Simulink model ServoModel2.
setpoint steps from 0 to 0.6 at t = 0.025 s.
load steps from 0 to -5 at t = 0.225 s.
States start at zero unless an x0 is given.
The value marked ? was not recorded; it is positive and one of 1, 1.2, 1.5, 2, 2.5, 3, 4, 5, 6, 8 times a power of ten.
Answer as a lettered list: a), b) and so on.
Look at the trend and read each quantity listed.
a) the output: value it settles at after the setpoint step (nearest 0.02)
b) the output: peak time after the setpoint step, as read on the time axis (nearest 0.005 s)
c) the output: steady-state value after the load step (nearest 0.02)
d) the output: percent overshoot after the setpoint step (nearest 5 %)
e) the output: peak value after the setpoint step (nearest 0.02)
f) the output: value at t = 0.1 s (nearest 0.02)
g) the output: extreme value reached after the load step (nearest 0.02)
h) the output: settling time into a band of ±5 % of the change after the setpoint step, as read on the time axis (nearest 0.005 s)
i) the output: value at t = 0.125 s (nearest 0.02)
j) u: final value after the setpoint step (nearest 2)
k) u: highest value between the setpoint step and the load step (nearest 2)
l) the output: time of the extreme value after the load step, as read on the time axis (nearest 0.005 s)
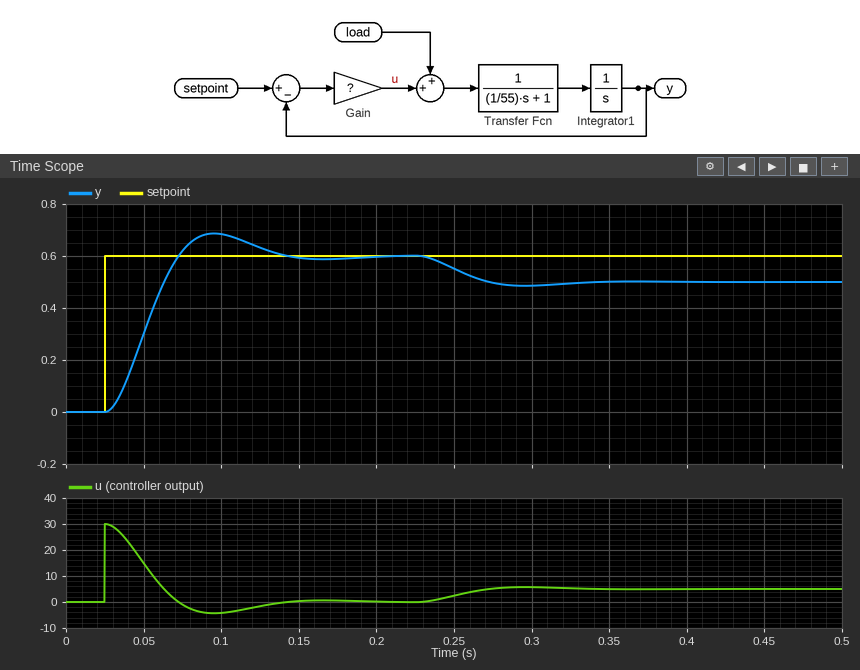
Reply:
a) 0.60
b) 0.095 s
c) 0.50
d) 15 %
e) 0.68
f) 0.68
g) 0.48
h) 0.125 s
i) 0.64
j) 0
k) 30
l) 0.295 s
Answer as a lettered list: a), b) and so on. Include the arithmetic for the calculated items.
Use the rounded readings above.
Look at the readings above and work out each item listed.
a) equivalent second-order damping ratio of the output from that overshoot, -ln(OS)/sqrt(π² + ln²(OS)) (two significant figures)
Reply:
a) ln(0.15) = -1.897; 1.897 / sqrt(9.870 + 3.599) = 0.52
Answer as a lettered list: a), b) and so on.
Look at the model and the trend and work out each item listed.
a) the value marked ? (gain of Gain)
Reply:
a) 50
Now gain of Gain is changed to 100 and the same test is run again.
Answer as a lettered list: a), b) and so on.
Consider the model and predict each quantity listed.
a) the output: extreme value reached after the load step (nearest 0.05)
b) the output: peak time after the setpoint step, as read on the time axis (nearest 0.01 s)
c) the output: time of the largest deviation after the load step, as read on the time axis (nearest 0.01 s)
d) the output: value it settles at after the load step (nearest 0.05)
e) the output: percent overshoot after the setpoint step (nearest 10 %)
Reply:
a) 0.55
b) 0.07 s
c) 0.27 s
d) 0.55
e) 30 %
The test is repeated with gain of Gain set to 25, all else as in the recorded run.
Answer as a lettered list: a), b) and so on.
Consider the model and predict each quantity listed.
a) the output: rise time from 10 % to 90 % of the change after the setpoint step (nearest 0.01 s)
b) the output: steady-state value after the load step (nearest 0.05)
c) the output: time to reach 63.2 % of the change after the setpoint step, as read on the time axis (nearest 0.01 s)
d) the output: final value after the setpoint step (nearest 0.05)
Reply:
a) 0.06 s
b) 0.40
c) 0.07 s
d) 0.60
